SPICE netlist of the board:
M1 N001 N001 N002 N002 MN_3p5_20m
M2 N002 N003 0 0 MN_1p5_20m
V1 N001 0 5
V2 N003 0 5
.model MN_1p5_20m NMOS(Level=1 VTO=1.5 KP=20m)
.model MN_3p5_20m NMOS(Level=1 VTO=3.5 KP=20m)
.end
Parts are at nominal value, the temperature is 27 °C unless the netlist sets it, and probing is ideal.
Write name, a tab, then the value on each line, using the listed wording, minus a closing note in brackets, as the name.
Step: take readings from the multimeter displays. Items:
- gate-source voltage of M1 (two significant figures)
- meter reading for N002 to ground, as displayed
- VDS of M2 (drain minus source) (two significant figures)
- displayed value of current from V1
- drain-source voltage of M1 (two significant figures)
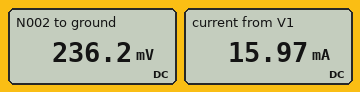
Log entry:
gate-source voltage of M1	4.8 V
meter reading for N002 to ground, as displayed	236.2 mV
VDS of M2 (drain minus source)	240 mV
displayed value of current from V1	15.97 mA
drain-source voltage of M1	4.8 V
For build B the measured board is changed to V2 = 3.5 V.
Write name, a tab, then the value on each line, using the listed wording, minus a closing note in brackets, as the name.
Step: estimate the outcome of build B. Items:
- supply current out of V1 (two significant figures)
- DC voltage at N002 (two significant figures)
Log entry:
supply current out of V1	13 mA
DC voltage at N002	360 mV
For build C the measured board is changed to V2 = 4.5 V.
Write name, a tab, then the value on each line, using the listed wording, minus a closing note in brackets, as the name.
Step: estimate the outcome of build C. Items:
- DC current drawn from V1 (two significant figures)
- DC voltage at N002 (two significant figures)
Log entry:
DC current drawn from V1	15 mA
DC voltage at N002	270 mV
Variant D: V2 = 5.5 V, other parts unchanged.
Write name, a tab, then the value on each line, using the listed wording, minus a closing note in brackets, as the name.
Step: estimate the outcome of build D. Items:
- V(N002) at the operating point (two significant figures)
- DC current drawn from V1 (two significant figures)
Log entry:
V(N002) at the operating point	210 mV
DC current drawn from V1	17 mA
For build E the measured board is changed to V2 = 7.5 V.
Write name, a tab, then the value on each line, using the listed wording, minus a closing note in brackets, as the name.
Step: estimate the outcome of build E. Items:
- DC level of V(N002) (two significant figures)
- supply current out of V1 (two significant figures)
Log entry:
DC level of V(N002)	150 mV
supply current out of V1	18 mA
